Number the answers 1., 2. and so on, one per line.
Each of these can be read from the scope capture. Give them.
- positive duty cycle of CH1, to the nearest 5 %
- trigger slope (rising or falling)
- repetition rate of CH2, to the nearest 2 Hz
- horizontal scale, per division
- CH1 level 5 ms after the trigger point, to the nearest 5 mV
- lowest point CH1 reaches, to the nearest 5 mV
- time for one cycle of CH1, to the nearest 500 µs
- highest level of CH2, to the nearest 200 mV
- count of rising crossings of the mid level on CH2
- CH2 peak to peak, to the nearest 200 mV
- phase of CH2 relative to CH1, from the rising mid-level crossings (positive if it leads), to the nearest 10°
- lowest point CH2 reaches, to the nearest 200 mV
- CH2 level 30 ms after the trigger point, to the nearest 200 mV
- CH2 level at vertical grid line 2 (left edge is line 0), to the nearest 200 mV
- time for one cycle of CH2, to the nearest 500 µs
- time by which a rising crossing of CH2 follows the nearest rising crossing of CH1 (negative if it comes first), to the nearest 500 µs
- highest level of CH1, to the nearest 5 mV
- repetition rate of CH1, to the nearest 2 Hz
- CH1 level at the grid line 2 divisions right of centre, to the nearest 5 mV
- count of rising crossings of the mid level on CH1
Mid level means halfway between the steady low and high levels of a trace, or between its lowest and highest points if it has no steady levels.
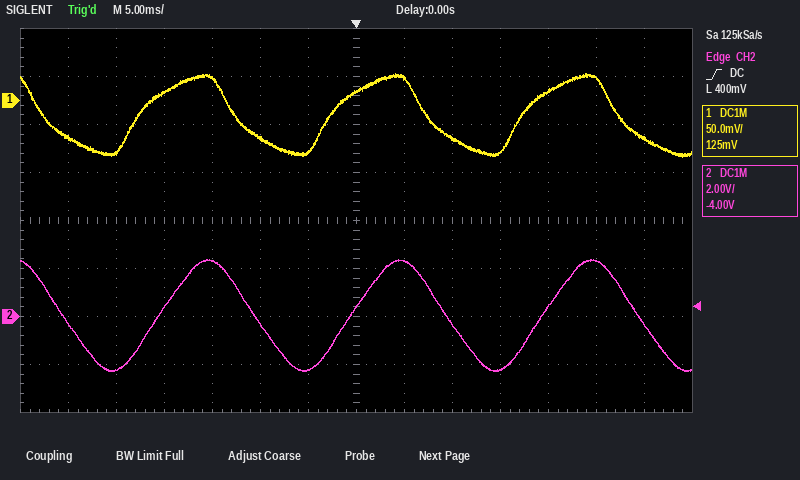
1. 50 %
2. rising
3. 50 Hz
4. 5 ms
5. 25 mV
6. -60 mV
7. 20.0 ms
8. 2.4 V
9. 3
10. 4.6 V
11. -40°
12. -2.2 V
13. -400 mV
14. -2.2 V
15. 20.0 ms
16. +2.0 ms
17. 30 mV
18. 50 Hz
19. -40 mV
20. 3
